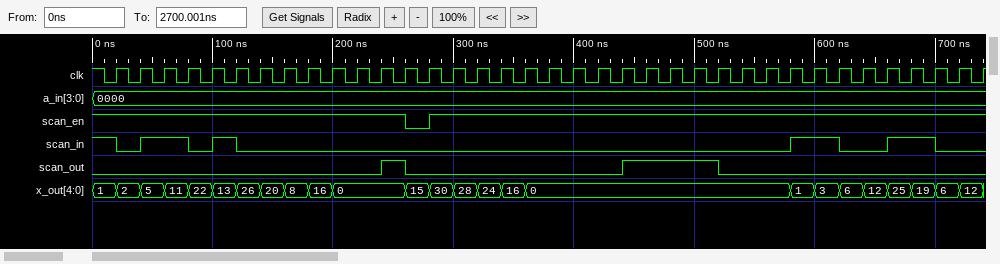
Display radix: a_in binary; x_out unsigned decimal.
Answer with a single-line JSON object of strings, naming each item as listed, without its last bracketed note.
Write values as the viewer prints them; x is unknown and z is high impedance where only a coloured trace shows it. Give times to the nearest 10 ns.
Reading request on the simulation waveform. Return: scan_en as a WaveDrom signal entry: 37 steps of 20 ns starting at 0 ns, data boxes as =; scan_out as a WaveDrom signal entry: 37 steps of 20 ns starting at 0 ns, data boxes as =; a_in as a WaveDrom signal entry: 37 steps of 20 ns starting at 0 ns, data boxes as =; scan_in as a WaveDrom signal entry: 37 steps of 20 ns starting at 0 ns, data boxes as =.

{"scan_en as a WaveDrom signal entry: 37 steps of 20 ns starting at 0 ns, data boxes as =": "{name: 'scan_en', wave: '1............01......................'}", "scan_out as a WaveDrom signal entry: 37 steps of 20 ns starting at 0 ns, data boxes as =": "{name: 'scan_out', wave: '0...........10........1...0..........'}", "a_in as a WaveDrom signal entry: 37 steps of 20 ns starting at 0 ns, data boxes as =": "{name: 'a_in', wave: '=....................................', data: '0000'}", "scan_in as a WaveDrom signal entry: 37 steps of 20 ns starting at 0 ns, data boxes as =": "{name: 'scan_in', wave: '101.010......................1.0.1.0.'}"}
